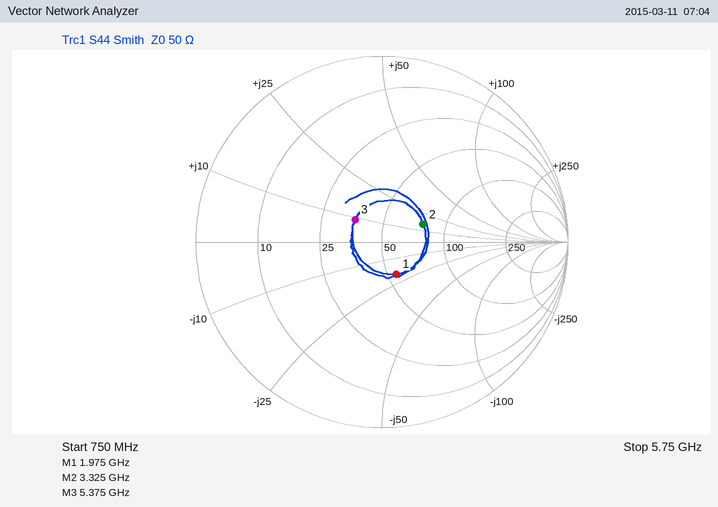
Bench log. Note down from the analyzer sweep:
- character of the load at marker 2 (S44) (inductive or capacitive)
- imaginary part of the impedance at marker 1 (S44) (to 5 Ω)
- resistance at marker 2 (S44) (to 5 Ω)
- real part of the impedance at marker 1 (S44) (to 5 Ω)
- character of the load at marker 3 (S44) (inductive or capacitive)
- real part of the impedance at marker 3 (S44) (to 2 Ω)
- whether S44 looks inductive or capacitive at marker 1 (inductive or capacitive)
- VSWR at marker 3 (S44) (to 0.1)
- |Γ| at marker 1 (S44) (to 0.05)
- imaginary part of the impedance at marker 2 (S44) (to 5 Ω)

inductive
-20 Ω
75 Ω
55 Ω
inductive
36 Ω
capacitive
1.5
0.20
+15 Ω
